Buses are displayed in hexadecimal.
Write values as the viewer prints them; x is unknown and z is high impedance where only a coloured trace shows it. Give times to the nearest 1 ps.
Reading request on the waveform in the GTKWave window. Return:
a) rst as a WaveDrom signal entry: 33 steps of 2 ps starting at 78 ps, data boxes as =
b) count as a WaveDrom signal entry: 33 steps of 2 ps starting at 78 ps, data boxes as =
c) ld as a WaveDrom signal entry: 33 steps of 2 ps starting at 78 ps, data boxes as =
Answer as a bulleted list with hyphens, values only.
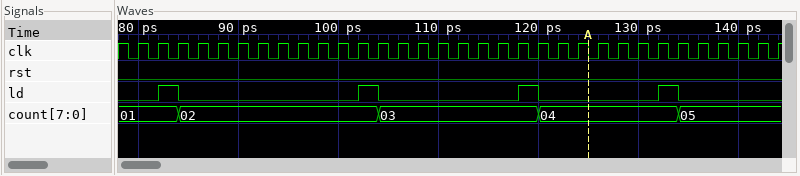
- {name: 'rst', wave: '0................................'}
- {name: 'count', wave: '=..=.........=.......=......=....', data: '01 02 03 04 05'}
- {name: 'ld', wave: '0.10........10......10.....10....'}
